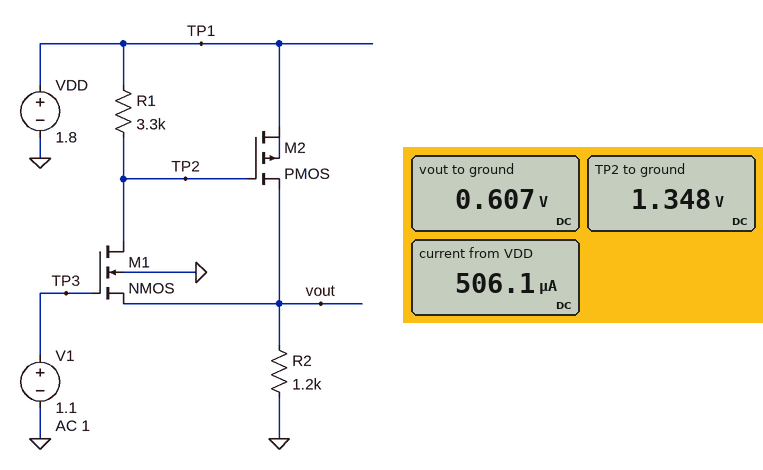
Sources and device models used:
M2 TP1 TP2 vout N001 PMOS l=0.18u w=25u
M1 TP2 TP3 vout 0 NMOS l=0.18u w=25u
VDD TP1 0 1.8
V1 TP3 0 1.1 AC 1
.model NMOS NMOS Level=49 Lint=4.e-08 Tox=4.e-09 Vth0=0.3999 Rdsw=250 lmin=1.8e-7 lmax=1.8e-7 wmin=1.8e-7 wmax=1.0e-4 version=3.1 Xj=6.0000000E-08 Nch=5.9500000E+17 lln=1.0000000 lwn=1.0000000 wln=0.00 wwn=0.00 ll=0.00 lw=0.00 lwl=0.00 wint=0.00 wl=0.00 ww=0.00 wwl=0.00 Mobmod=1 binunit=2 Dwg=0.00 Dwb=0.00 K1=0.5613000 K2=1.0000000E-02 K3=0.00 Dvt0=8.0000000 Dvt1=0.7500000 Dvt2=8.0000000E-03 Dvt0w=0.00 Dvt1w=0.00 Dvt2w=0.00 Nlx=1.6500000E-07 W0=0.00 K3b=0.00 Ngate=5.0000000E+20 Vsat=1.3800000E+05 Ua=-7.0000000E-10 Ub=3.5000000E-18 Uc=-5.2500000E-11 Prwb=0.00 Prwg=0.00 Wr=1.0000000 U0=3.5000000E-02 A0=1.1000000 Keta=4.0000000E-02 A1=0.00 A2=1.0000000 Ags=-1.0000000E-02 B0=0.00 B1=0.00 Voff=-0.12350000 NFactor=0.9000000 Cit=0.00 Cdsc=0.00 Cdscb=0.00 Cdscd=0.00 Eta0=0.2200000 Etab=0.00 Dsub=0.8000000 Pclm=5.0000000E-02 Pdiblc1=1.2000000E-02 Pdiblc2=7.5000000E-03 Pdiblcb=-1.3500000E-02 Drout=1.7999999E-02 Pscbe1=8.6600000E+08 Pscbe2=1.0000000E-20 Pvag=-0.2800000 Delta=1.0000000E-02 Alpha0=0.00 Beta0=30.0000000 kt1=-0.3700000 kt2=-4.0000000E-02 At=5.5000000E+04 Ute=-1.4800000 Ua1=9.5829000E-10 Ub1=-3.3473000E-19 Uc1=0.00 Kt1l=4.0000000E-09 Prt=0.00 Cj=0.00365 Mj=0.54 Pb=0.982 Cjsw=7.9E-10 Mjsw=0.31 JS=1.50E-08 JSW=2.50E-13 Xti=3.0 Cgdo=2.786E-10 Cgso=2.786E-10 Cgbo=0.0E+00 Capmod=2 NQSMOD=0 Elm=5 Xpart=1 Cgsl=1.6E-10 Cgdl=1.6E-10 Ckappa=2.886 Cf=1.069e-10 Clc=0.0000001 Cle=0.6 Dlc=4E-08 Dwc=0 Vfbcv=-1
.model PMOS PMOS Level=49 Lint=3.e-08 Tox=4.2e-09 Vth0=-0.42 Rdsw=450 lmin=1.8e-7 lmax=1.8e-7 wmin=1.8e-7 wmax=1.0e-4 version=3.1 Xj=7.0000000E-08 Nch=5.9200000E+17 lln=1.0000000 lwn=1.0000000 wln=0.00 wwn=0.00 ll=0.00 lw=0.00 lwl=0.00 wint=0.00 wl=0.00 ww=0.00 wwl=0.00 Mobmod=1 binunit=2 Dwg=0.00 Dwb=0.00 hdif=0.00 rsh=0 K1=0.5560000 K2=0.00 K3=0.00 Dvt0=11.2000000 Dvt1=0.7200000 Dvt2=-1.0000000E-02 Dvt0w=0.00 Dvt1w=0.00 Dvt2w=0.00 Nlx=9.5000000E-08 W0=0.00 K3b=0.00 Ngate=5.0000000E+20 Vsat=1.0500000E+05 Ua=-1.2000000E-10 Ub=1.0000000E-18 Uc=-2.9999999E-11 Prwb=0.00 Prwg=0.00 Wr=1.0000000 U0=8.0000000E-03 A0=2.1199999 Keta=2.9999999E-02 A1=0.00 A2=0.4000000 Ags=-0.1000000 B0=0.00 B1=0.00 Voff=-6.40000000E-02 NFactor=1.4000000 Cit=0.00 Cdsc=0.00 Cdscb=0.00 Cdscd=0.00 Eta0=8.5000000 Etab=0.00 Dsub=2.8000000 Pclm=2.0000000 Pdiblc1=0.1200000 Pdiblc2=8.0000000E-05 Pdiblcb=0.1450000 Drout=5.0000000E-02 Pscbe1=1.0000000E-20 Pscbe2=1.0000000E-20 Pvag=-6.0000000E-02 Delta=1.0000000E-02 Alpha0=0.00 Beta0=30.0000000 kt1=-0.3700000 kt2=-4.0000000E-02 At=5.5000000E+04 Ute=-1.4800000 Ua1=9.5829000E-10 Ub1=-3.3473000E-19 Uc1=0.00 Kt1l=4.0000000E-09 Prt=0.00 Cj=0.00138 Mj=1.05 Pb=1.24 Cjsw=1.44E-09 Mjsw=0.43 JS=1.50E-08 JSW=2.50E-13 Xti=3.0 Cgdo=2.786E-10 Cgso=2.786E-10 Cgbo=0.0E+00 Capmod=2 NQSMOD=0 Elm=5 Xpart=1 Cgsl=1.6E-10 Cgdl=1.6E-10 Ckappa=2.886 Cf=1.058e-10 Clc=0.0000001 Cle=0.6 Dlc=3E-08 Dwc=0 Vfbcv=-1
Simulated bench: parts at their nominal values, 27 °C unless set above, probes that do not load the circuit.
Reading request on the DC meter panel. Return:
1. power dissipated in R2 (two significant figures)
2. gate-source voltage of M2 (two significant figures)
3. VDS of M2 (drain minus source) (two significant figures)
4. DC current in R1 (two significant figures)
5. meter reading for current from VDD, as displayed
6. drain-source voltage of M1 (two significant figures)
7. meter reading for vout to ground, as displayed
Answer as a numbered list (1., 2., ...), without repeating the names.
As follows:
1. 310 µW
2. 740 mV
3. 1.2 V
4. 140 µA
5. 506.1 µA
6. 740 mV
7. 0.607 V
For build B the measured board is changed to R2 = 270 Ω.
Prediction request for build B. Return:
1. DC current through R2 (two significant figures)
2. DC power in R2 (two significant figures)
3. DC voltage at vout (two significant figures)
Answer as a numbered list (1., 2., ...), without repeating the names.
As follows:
1. 2.1 mA
2. 1.2 mW
3. 560 mV
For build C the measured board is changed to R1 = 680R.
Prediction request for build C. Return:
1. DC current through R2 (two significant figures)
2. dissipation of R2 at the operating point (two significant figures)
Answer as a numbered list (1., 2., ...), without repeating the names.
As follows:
1. 460 µA
2. 260 µW
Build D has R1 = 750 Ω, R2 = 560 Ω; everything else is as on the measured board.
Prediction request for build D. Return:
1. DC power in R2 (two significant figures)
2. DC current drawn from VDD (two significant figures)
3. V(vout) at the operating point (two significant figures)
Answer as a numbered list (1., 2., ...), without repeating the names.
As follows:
1. 490 µW
2. 930 µA
3. 520 mV
